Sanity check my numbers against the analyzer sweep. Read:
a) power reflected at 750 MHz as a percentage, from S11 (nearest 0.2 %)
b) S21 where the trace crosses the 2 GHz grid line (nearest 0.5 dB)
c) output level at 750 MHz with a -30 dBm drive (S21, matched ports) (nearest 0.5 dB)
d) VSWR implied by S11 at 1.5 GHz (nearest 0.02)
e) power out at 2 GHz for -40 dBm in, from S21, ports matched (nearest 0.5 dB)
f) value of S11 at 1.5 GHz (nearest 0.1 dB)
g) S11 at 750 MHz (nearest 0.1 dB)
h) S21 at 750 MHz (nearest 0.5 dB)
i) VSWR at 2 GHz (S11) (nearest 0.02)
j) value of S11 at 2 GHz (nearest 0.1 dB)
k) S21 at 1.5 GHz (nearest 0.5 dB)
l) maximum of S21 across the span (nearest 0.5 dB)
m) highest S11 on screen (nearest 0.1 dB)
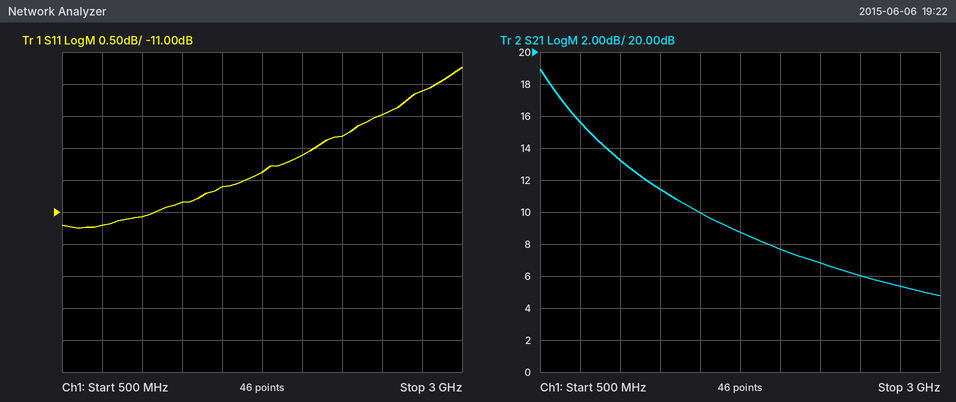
7.6 %
7.5 dB
-14.5 dBm
1.84
-32.5 dBm
-10.6 dB
-11.2 dB
15.5 dB
1.90
-10.1 dB
10.0 dB
19.0 dB
-8.7 dB
